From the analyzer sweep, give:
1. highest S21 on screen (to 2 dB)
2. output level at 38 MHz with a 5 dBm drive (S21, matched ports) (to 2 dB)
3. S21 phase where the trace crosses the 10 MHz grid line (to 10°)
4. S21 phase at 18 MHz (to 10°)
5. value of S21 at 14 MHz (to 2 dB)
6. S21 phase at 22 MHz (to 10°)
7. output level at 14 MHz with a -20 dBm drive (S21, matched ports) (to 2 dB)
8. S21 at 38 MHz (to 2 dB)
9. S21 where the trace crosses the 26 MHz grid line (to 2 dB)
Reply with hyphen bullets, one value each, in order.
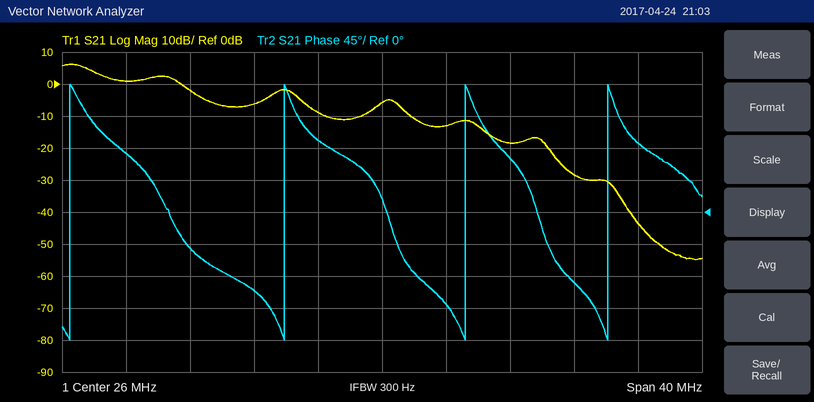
- 6 dB
- -24 dBm
- 80°
- -110°
- -2 dB
- 100°
- -22 dBm
- -28 dB
- -6 dB
